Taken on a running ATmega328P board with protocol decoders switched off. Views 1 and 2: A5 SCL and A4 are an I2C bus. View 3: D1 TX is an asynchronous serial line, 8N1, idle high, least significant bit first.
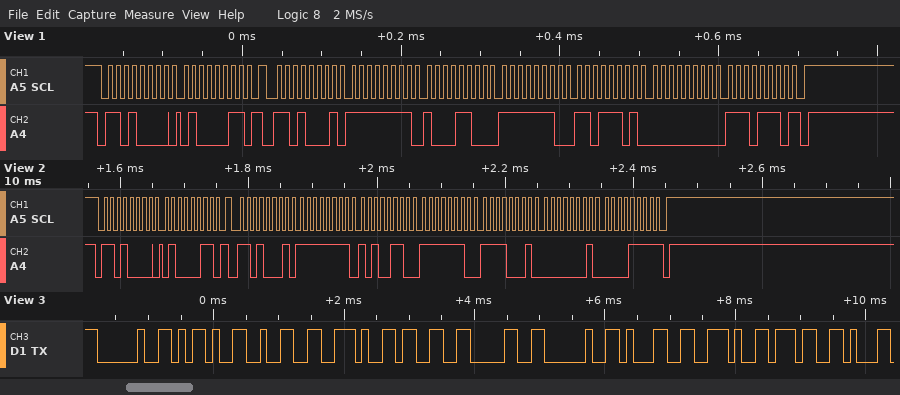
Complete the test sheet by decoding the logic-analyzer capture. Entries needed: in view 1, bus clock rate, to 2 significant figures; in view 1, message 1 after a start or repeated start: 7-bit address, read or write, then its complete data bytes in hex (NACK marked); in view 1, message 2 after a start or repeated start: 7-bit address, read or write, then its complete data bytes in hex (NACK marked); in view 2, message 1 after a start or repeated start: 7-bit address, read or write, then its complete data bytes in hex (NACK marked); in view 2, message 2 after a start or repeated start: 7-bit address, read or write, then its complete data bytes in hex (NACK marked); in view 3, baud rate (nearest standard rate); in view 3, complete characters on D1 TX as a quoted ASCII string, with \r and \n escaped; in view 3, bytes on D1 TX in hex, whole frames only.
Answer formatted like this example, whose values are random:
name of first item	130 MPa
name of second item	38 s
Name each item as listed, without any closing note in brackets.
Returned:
in view 1, bus clock rate, to 2 significant figures	100 kHz
in view 1, message 1 after a start or repeated start: 7-bit address, read or write, then its complete data bytes in hex	0x68 write: 43
in view 1, message 2 after a start or repeated start: 7-bit address, read or write, then its complete data bytes in hex	0x68 read: FF 8C FE DD 00 EE NACK
in view 2, message 1 after a start or repeated start: 7-bit address, read or write, then its complete data bytes in hex	0x68 write: 43
in view 2, message 2 after a start or repeated start: 7-bit address, read or write, then its complete data bytes in hex	0x68 read: FF A6 FE F1 01 0F NACK
in view 3, baud rate	9600 baud
in view 3, complete characters on D1 TX as a quoted ASCII string, with \r and \n escaped	" -2.30 1.7"
in view 3, bytes on D1 TX in hex, whole frames only	20 2D 32 2E 33 30 20 31 2E 37
